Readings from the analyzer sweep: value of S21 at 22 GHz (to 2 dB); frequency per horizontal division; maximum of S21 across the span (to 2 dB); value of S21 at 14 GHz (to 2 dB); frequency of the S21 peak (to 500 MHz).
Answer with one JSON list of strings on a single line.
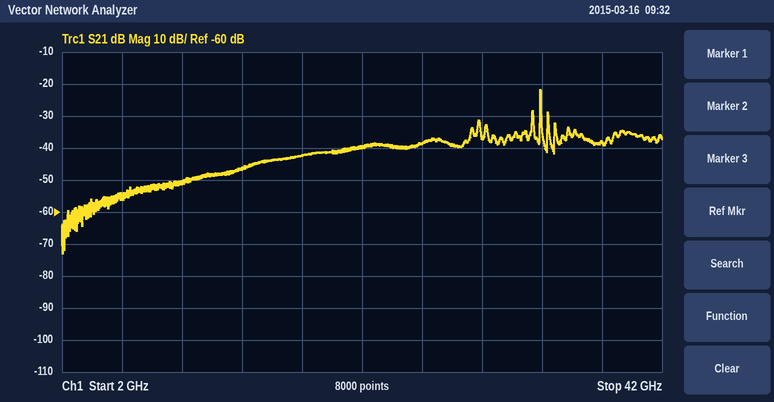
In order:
["-40 dB", "4 GHz", "-22 dB", "-46 dB", "34.0 GHz"]
